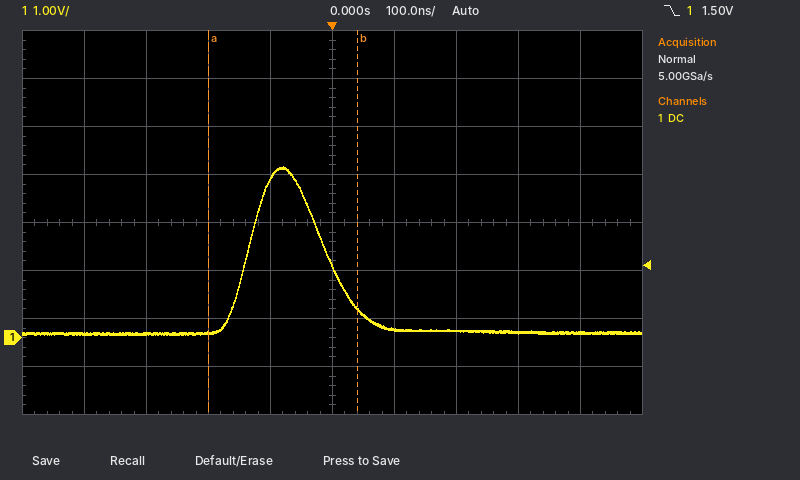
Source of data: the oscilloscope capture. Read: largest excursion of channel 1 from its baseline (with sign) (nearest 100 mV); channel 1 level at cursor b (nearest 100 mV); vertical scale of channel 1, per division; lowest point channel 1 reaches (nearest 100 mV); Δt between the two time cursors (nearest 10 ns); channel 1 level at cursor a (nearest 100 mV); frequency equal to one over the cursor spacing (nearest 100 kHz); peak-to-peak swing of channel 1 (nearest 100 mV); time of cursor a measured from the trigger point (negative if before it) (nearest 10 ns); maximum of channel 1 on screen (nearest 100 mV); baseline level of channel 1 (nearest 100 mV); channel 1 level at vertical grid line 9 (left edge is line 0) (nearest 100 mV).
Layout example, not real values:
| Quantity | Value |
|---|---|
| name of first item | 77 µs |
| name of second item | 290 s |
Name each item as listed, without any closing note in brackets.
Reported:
| Quantity | Value |
|---|---|
| largest excursion of channel 1 from its baseline (with sign) | +3.5 V |
| channel 1 level at cursor b | 600 mV |
| vertical scale of channel 1, per division | 1 V |
| lowest point channel 1 reaches | 100 mV |
| Δt between the two time cursors | 240 ns |
| channel 1 level at cursor a | 100 mV |
| frequency equal to one over the cursor spacing | 4.2 MHz |
| peak-to-peak swing of channel 1 | 3.5 V |
| time of cursor a measured from the trigger point (negative if before it) | -200 ns |
| maximum of channel 1 on screen | 3.6 V |
| baseline level of channel 1 | 100 mV |
| channel 1 level at vertical grid line 9 (left edge is line 0) | 100 mV |
